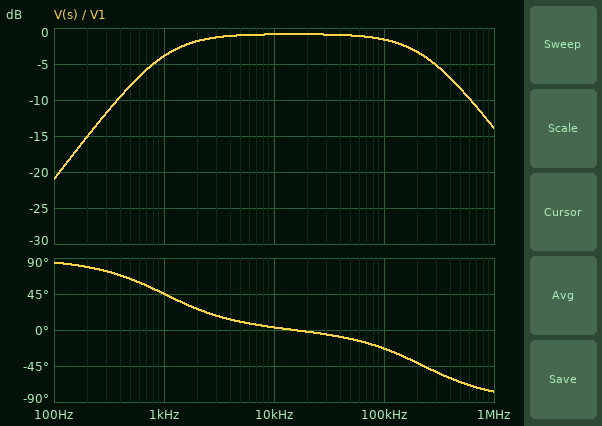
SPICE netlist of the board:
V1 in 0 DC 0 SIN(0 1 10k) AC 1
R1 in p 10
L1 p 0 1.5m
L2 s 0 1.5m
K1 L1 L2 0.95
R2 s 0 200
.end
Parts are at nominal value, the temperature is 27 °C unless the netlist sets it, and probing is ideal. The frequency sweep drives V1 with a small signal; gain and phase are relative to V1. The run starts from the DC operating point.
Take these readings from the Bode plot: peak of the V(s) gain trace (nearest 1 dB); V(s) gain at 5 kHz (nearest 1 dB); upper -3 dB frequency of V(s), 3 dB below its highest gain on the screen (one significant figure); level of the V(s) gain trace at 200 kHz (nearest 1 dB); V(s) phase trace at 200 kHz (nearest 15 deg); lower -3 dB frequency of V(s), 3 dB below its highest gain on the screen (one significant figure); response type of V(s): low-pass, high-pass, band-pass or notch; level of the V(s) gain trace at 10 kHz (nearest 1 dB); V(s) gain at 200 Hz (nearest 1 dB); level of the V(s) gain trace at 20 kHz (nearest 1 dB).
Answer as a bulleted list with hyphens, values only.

- -1 dB
- -1 dB
- 200 kHz
- -3 dB
- -45 deg
- 1 kHz
- band-pass
- -1 dB
- -15 dB
- -1 dB
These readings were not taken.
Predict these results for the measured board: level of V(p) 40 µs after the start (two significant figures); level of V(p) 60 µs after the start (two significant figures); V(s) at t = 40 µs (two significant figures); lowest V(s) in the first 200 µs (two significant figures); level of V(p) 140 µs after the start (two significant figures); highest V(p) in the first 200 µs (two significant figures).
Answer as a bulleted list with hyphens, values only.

- 400 mV
- -700 mV
- 420 mV
- -960 mV
- 440 mV
- 910 mV
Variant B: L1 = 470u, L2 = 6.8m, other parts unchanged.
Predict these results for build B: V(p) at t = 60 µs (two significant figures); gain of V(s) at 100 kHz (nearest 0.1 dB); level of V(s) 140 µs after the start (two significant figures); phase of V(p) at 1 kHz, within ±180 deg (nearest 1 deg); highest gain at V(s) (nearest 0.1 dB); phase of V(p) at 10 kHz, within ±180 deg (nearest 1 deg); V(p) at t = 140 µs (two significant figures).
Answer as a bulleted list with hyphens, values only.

- -520 mV
- 2.6 dB
- 1.0 V
- 64 deg
- 6.4 dB
- 16 deg
- 180 mV
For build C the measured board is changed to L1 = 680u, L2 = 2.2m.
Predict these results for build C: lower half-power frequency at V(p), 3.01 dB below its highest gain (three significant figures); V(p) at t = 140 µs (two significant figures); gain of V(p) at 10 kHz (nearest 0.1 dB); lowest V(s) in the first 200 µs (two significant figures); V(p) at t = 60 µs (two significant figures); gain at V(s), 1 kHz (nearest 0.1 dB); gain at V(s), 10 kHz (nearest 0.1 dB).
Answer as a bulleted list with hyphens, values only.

- 2.83 kHz
- 320 mV
- -1.4 dB
- -1.6 V
- -710 mV
- -3.7 dB
- 3.3 dB
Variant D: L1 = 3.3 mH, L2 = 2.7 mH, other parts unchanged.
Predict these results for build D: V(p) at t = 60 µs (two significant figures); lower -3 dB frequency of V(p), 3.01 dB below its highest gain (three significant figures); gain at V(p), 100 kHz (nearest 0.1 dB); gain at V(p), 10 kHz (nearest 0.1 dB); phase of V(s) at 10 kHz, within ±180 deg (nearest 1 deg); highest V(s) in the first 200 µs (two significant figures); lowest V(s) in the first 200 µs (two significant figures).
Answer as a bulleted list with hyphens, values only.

- -640 mV
- 502 Hz
- -0.2 dB
- -0.3 dB
- -2 deg
- 800 mV
- -860 mV
